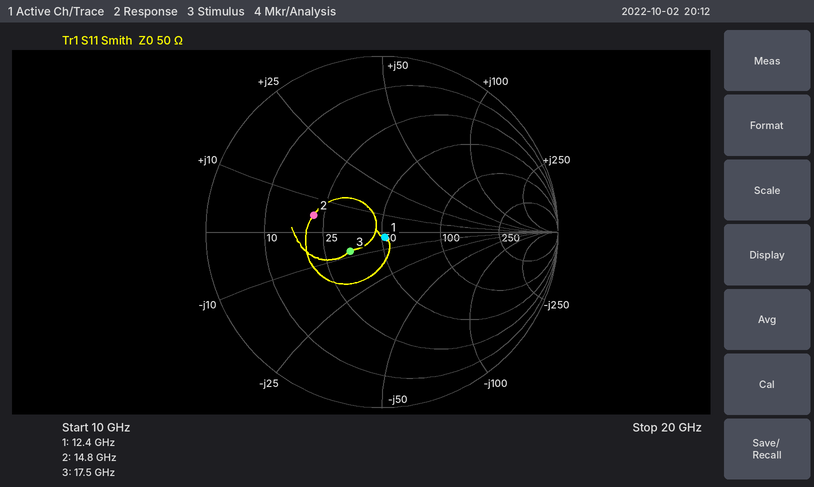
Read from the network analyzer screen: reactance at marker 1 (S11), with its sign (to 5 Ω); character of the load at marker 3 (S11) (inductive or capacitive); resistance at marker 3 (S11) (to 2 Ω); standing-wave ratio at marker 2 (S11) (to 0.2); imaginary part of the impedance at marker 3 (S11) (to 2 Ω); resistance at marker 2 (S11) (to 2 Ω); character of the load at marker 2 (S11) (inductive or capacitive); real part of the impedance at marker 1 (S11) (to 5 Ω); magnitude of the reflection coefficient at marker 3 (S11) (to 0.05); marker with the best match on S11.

-5 Ω
capacitive
34 Ω
2.4
-8 Ω
22 Ω
inductive
50 Ω
0.20
marker 1
